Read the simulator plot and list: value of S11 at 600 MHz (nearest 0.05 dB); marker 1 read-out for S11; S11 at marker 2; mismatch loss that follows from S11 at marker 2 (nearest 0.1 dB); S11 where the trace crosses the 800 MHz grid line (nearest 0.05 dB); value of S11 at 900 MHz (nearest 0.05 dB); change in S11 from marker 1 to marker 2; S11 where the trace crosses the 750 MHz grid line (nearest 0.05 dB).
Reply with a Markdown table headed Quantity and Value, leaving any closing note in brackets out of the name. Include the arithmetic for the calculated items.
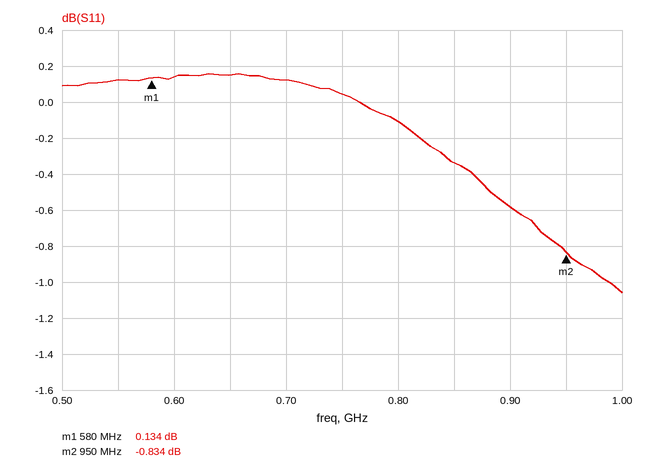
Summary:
| Quantity | Value |
|---|---|
| value of S11 at 600 MHz | 0.15 dB |
| marker 1 read-out for S11 | 0.134 dB |
| S11 at marker 2 | -0.834 dB |
| mismatch loss that follows from S11 at marker 2 | −10 log10(1 − 10^(-0.834/10)) ≈ 7.6 dB |
| S11 where the trace crosses the 800 MHz grid line | -0.10 dB |
| value of S11 at 900 MHz | -0.60 dB |
| change in S11 from marker 1 to marker 2 | -0.834 − (0.134) = -0.968 dB |
| S11 where the trace crosses the 750 MHz grid line | 0.05 dB |
